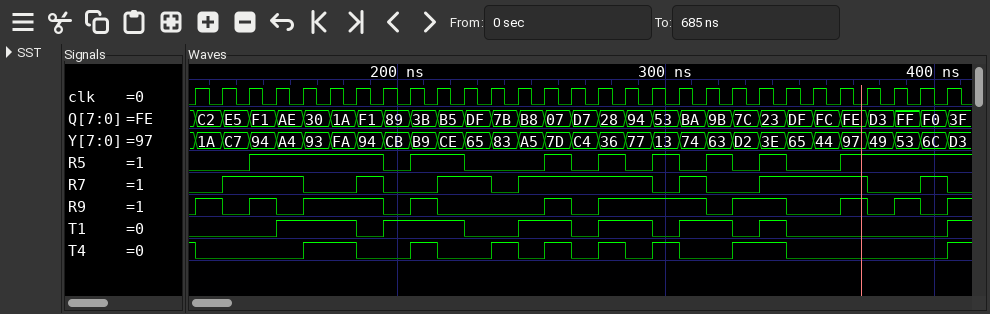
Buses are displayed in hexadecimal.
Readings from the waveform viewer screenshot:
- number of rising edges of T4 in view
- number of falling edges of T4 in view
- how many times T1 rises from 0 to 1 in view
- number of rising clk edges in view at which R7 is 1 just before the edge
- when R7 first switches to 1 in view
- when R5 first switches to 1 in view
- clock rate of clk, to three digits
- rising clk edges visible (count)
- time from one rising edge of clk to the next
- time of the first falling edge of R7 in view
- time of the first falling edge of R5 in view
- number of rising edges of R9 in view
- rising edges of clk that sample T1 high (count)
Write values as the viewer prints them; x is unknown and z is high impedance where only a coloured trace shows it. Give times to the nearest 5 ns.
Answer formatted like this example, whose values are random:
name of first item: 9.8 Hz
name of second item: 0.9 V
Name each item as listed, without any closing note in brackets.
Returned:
number of rising edges of T4 in view: 8
number of falling edges of T4 in view: 8
how many times T1 rises from 0 to 1 in view: 7
number of rising clk edges in view at which R7 is 1 just before the edge: 17
when R7 first switches to 1 in view: 135 ns
when R5 first switches to 1 in view: 145 ns
clock rate of clk, to three digits: 100 MHz
rising clk edges visible: 29
time from one rising edge of clk to the next: 10 ns
time of the first falling edge of R7 in view: 165 ns
time of the first falling edge of R5 in view: 195 ns
number of rising edges of R9 in view: 10
rising edges of clk that sample T1 high: 13
